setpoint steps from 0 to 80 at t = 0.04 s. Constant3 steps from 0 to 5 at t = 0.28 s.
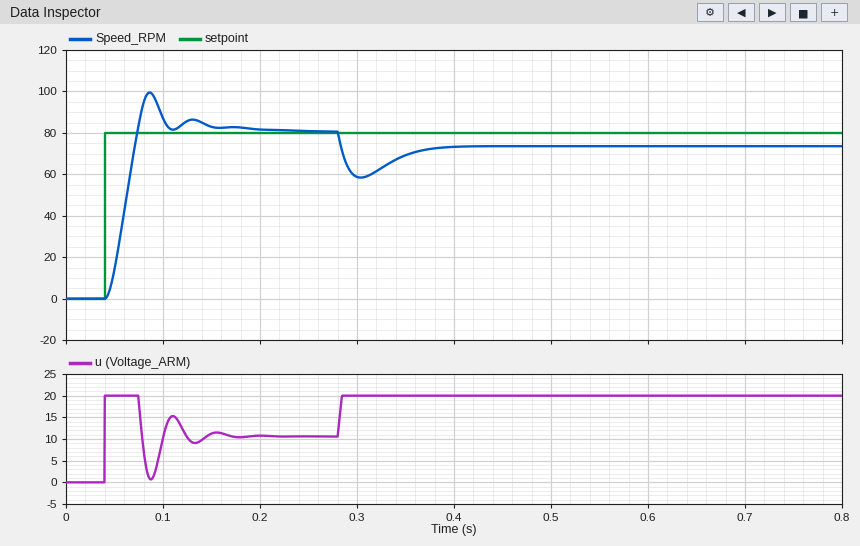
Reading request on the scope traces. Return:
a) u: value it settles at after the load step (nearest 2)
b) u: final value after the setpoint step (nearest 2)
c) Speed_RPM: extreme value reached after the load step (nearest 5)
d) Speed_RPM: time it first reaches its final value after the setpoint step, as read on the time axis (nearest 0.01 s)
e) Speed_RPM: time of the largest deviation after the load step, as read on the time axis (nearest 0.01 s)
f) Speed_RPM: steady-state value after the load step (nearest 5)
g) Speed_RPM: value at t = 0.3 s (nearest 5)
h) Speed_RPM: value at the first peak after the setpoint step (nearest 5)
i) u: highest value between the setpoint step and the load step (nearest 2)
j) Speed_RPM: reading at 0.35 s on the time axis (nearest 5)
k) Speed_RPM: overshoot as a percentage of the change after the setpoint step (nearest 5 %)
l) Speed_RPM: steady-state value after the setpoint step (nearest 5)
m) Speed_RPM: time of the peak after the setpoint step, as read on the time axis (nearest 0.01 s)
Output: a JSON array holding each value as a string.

["20", "10", "60", "0.07 s", "0.30 s", "75", "60", "100", "20", "70", "25 %", "80", "0.09 s"]
